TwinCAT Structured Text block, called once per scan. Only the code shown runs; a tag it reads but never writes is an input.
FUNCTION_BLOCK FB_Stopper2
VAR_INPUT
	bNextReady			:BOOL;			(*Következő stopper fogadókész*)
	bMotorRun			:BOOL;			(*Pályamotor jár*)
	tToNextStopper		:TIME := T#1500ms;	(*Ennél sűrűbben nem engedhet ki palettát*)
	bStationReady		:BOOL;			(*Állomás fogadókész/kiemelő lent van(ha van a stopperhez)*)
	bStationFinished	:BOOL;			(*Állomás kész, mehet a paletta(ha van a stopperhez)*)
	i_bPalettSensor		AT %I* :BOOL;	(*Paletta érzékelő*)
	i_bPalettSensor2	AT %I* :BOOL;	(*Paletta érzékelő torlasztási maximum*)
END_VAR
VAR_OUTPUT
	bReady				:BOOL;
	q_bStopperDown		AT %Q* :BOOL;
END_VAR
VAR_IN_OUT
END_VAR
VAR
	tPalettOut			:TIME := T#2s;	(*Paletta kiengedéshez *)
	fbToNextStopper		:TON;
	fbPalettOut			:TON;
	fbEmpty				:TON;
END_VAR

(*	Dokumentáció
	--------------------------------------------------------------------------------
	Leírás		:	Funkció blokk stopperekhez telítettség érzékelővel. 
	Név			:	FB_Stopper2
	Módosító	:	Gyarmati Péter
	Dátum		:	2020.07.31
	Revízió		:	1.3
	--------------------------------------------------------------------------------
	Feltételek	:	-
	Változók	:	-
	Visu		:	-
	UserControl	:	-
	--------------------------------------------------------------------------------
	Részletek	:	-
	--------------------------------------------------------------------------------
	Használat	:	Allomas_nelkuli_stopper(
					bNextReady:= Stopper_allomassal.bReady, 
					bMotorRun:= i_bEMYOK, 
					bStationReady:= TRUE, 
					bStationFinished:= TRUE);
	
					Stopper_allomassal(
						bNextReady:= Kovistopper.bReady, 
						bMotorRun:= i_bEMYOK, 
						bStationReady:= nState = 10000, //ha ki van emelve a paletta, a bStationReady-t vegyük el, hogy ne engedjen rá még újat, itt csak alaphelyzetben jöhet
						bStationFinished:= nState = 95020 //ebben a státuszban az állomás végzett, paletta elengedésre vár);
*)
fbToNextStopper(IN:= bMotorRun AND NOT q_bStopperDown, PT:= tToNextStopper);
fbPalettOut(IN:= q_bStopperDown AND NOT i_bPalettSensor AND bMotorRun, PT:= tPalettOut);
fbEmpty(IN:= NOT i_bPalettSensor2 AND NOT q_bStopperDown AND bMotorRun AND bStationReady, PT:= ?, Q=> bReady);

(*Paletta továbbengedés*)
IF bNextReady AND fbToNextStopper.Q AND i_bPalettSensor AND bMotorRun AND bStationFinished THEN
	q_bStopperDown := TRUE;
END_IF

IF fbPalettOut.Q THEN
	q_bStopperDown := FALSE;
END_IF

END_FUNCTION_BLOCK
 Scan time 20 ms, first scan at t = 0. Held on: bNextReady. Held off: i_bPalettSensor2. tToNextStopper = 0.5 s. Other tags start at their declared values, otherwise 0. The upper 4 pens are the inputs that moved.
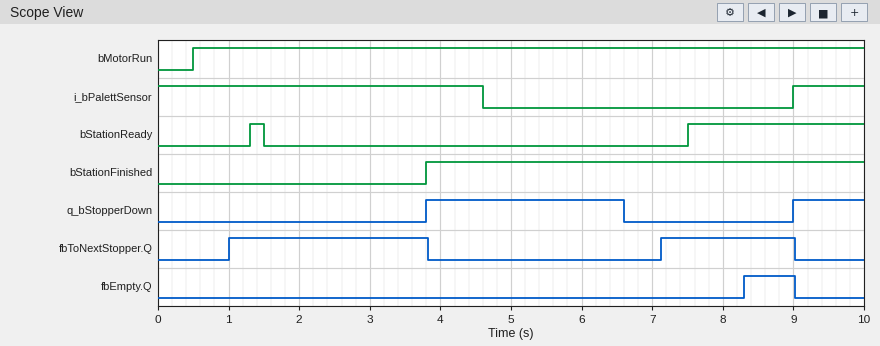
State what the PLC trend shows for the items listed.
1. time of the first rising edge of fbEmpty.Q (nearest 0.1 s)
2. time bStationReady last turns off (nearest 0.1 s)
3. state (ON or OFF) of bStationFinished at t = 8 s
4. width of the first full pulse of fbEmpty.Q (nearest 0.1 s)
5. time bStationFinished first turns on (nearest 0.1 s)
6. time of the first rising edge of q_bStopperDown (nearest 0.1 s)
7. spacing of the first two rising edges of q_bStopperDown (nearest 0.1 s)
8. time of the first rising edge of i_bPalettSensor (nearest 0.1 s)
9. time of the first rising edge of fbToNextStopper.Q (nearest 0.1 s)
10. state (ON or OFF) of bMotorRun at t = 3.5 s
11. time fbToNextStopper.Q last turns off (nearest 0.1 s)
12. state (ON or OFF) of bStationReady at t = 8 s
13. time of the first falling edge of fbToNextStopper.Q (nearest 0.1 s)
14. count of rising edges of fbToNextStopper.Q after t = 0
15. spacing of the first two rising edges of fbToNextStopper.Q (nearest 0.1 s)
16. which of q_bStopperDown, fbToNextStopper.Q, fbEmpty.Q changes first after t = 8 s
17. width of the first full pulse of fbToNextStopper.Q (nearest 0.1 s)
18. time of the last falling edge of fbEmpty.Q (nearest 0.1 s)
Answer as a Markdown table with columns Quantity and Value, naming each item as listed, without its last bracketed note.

| Quantity | Value |
|---|---|
| time of the first rising edge of fbEmpty.Q | 8.3 s |
| time bStationReady last turns off | 1.5 s |
| state (ON or OFF) of bStationFinished at t = 8 s | ON |
| width of the first full pulse of fbEmpty.Q | 0.7 s |
| time bStationFinished first turns on | 3.8 s |
| time of the first rising edge of q_bStopperDown | 3.8 s |
| spacing of the first two rising edges of q_bStopperDown | 5.2 s |
| time of the first rising edge of i_bPalettSensor | 9.0 s |
| time of the first rising edge of fbToNextStopper.Q | 1.0 s |
| state (ON or OFF) of bMotorRun at t = 3.5 s | ON |
| time fbToNextStopper.Q last turns off | 9.0 s |
| state (ON or OFF) of bStationReady at t = 8 s | ON |
| time of the first falling edge of fbToNextStopper.Q | 3.8 s |
| count of rising edges of fbToNextStopper.Q after t = 0 | 2 |
| spacing of the first two rising edges of fbToNextStopper.Q | 6.1 s |
| which of q_bStopperDown, fbToNextStopper.Q, fbEmpty.Q changes first after t = 8 s | fbEmpty.Q |
| width of the first full pulse of fbToNextStopper.Q | 2.8 s |
| time of the last falling edge of fbEmpty.Q | 9.0 s |
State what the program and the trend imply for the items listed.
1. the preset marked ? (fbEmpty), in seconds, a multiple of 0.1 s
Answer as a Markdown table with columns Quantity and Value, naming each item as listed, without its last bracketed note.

| Quantity | Value |
|---|---|
| the preset marked ? (fbEmpty), in seconds, a multiple of 0.1 s | 0.8 s |
